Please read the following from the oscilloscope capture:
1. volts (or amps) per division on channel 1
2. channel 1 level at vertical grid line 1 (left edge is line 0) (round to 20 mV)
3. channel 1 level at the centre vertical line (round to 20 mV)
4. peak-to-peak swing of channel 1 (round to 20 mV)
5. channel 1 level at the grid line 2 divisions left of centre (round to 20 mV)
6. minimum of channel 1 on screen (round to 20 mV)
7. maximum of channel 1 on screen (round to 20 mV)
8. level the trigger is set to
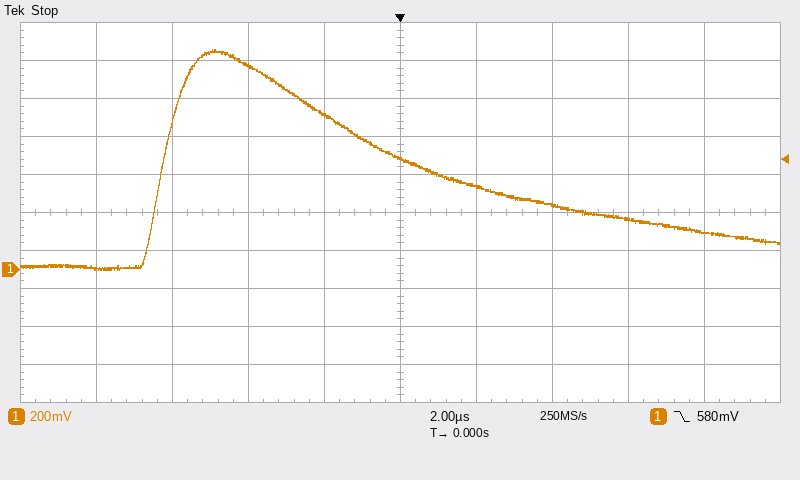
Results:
200 mV
0 mV
580 mV
1.16 V
1.08 V
0 mV
1.16 V
580 mV
